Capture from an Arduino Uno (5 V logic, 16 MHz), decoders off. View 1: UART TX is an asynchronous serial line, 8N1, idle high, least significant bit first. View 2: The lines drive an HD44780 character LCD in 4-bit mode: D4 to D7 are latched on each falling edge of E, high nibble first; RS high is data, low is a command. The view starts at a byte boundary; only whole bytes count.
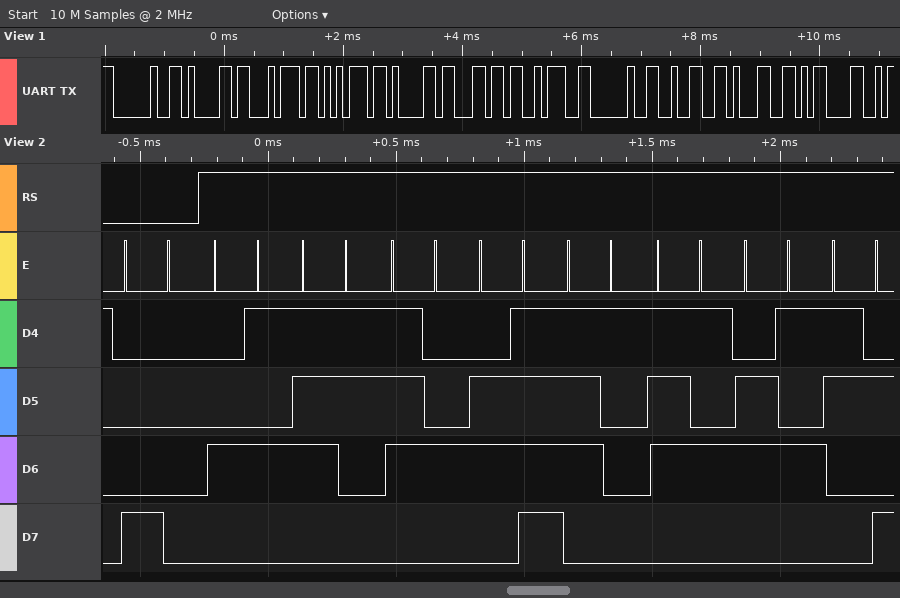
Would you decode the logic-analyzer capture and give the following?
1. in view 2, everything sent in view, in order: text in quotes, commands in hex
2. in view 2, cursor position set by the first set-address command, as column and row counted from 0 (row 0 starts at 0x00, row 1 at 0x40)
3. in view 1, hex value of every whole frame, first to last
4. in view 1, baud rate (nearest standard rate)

0x80 "Estoque:"
column 0, row 0
0x20 0x61 0x74 0x75 0x61 0x6C 0x3A 0x20 0x32 0x31 0x0D
9600 baud
